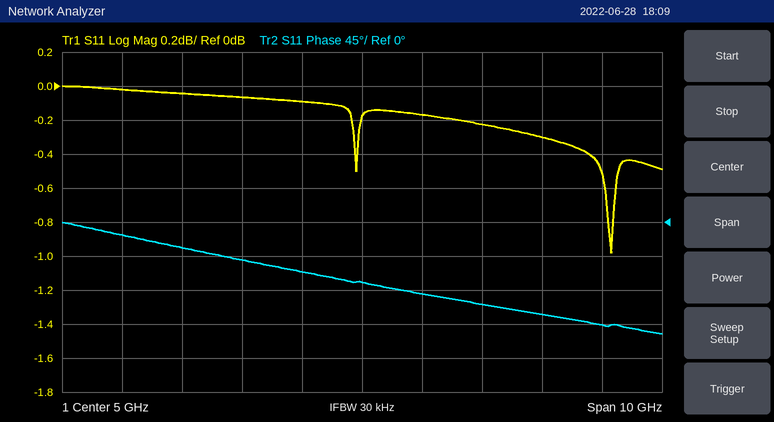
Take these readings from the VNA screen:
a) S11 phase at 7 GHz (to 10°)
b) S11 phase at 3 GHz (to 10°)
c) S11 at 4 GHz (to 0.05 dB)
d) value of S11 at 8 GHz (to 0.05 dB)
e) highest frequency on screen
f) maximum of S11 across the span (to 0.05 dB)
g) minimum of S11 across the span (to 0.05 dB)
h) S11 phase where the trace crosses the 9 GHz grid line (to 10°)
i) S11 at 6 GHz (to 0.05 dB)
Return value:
-110°
-50°
-0.10 dB
-0.30 dB
10 GHz
0.00 dB
-1.00 dB
-140°
-0.15 dB
